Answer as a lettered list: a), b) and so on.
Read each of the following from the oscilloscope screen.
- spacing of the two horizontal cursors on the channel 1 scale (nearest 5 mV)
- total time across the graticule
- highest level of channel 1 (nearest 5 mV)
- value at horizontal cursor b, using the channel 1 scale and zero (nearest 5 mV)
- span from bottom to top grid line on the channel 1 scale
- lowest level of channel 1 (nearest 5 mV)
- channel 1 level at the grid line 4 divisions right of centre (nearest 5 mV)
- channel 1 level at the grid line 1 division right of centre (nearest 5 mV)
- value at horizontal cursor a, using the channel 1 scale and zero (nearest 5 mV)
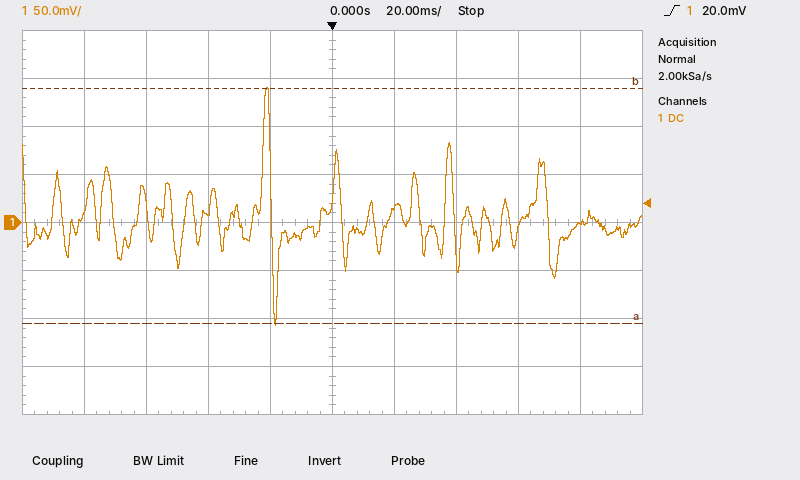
a) 245 mV
b) 200 ms
c) 140 mV
d) 140 mV
e) 400 mV
f) -105 mV
g) 0 mV
h) 15 mV
i) -105 mV
